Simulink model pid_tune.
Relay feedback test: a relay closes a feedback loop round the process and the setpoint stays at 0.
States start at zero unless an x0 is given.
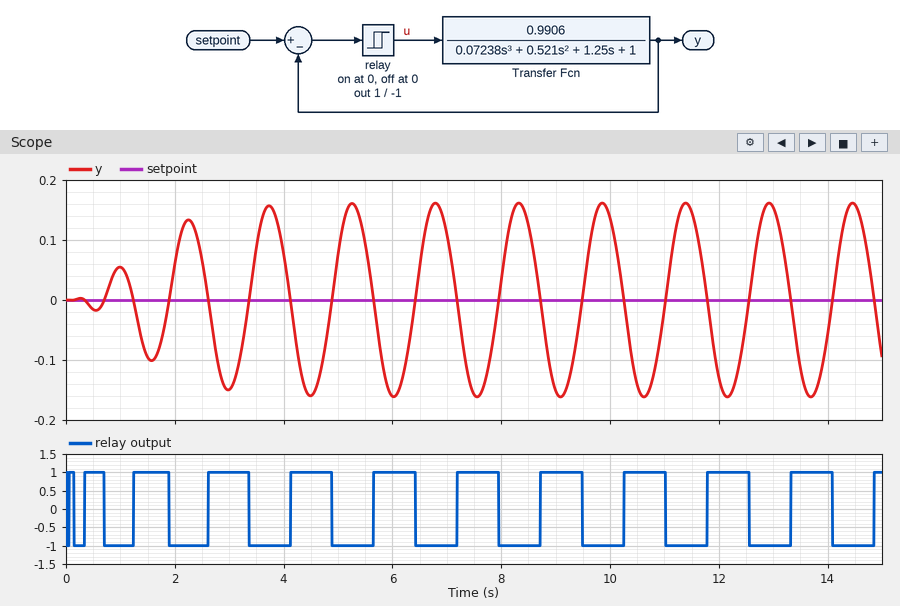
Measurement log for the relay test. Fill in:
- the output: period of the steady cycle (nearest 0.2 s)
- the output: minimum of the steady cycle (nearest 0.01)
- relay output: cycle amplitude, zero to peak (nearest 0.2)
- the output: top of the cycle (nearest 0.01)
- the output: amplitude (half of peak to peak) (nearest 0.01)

1.6 s
-0.16
1.0
0.16
0.16
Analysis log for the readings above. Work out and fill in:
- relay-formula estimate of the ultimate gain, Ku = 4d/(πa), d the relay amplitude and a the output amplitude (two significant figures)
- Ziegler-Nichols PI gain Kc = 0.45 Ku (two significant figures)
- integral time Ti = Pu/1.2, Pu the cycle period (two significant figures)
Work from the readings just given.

8.0
3.6
1.3 s
